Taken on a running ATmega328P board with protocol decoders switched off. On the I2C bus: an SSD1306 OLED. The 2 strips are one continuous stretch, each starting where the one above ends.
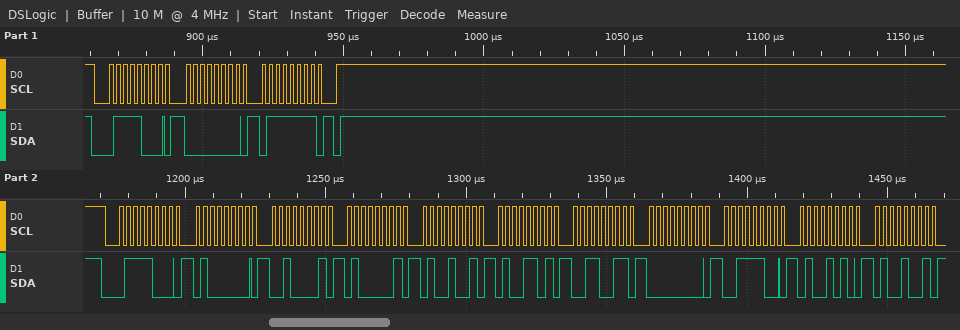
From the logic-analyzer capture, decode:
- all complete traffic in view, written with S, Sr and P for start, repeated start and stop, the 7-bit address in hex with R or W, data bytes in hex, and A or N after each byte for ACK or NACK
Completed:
S 3CW A 00 A 7F A P S 3CW A 40 A 21 A 41 A 49 A 4D A 33 A 00 A 3C A 4A A 49 A
